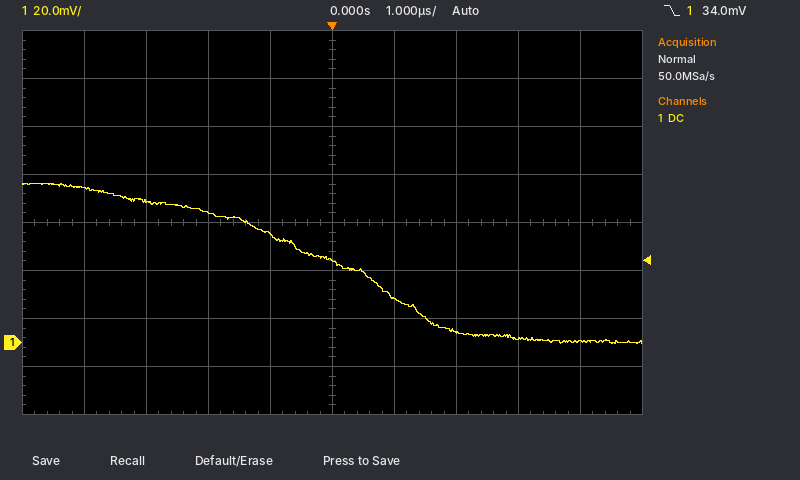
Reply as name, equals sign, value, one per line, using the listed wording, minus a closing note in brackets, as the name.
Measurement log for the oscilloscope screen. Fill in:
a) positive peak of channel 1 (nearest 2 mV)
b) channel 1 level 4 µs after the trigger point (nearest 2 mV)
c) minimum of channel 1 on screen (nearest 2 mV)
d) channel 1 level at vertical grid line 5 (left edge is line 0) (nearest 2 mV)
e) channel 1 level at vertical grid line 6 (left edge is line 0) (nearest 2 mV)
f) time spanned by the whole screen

positive peak of channel 1 = 66 mV
channel 1 level 4 µs after the trigger point = 0 mV
minimum of channel 1 on screen = 0 mV
channel 1 level at vertical grid line 5 (left edge is line 0) = 34 mV
channel 1 level at vertical grid line 6 (left edge is line 0) = 18 mV
time spanned by the whole screen = 10 µs
